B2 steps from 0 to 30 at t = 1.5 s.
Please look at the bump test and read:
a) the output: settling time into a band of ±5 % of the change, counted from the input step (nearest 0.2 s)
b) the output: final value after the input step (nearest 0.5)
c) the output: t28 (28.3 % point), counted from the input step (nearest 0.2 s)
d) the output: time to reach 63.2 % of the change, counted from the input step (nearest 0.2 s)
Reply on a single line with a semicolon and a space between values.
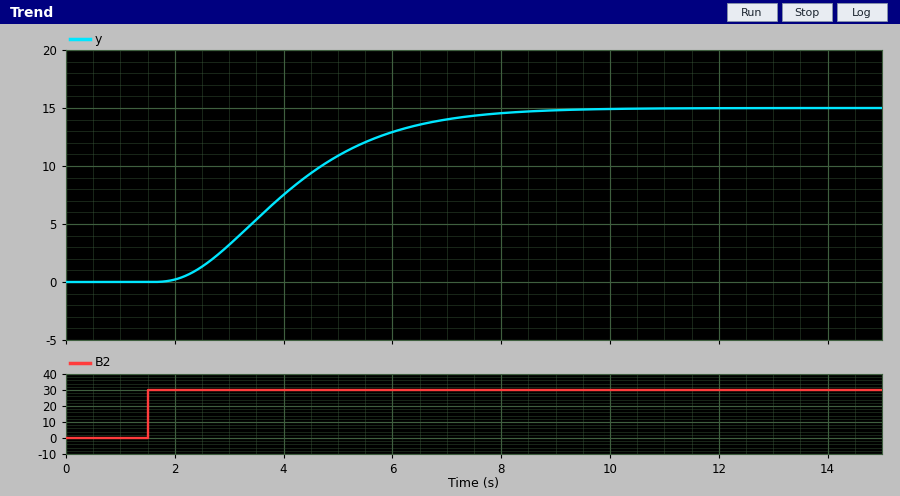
5.8 s; 15.0; 1.8 s; 3.0 s
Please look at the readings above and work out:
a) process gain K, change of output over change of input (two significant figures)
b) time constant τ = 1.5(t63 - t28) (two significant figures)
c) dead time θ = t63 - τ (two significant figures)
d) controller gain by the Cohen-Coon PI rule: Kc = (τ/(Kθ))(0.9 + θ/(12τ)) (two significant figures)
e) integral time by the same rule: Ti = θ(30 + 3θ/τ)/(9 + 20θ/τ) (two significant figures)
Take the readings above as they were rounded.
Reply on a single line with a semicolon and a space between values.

0.50; 1.8 s; 1.2 s; 2.9; 1.7 s
